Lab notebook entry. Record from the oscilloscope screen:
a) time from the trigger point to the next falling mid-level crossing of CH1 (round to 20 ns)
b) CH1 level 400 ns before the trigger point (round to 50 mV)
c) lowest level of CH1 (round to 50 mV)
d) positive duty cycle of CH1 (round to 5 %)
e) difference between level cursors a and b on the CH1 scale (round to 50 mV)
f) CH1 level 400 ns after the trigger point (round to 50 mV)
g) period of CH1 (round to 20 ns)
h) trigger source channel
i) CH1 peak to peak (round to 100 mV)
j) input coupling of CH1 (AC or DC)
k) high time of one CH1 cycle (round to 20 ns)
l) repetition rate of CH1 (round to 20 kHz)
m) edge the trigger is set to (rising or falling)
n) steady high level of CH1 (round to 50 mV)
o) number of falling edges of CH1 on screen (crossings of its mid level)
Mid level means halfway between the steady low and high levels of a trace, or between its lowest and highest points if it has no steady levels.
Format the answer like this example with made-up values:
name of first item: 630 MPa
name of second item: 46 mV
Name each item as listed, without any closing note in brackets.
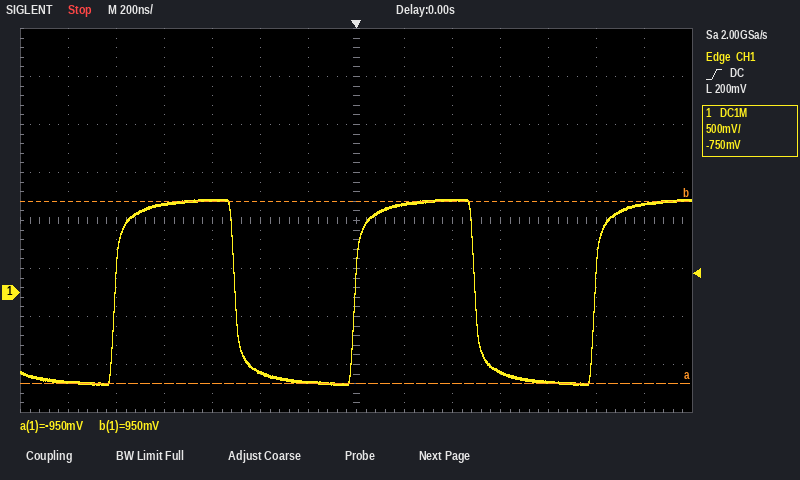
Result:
time from the trigger point to the next falling mid-level crossing of CH1: 500 ns
CH1 level 400 ns before the trigger point: -850 mV
lowest level of CH1: -950 mV
positive duty cycle of CH1: 50 %
difference between level cursors a and b on the CH1 scale: 1.90 V
CH1 level 400 ns after the trigger point: 950 mV
period of CH1: 1.00 µs
trigger source channel: CH1
CH1 peak to peak: 1.90 V
input coupling of CH1: DC
high time of one CH1 cycle: 500 ns
repetition rate of CH1: 1.00 MHz
edge the trigger is set to: rising
steady high level of CH1: 950 mV
number of falling edges of CH1 on screen: 2
